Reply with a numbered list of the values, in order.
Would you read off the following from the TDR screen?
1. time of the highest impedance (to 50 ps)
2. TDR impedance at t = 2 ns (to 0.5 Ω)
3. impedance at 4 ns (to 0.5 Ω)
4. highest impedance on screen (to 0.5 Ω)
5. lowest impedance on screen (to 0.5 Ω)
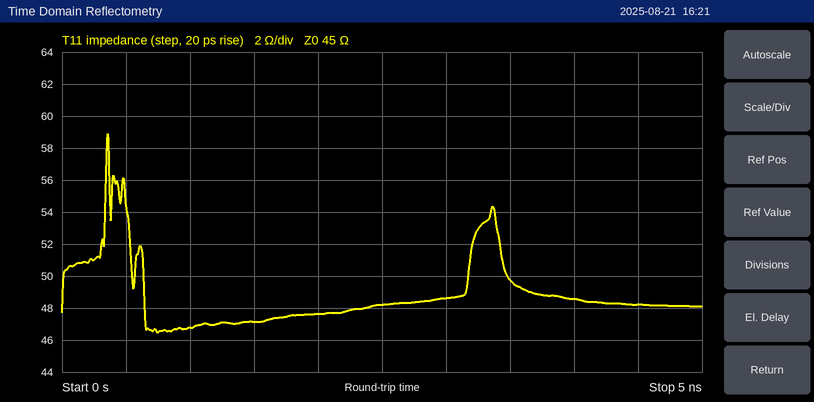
1. 350 ps
2. 47.5 Ω
3. 48.5 Ω
4. 59.0 Ω
5. 46.5 Ω
